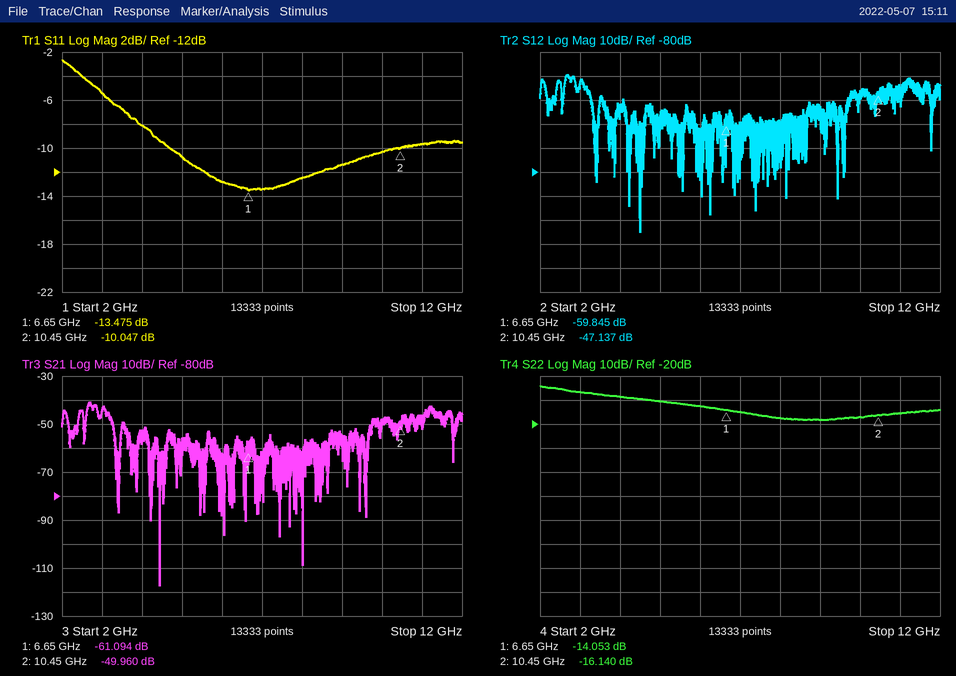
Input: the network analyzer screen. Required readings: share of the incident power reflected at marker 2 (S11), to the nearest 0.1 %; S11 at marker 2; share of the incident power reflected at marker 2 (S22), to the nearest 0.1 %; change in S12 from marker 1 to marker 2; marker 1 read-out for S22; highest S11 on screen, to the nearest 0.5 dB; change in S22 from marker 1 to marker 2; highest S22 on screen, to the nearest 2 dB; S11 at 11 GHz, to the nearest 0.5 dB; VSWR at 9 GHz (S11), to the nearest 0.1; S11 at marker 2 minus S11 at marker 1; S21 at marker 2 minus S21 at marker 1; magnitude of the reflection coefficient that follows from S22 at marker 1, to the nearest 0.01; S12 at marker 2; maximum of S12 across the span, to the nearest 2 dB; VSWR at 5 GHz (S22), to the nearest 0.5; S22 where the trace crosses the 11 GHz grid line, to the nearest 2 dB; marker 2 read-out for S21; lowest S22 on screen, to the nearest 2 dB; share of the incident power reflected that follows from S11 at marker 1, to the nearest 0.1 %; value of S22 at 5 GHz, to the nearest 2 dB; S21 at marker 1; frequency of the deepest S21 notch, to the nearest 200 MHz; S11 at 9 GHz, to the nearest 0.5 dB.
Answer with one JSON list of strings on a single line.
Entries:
["9.9 %", "-10.047 dB", "2.4 %", "12.708 dB", "-14.053 dB", "-2.5 dB", "-2.087 dB", "-4 dB", "-9.5 dB", "1.7", "3.428 dB", "11.134 dB", "0.20", "-47.137 dB", "-40 dB", "2.0", "-16 dB", "-49.960 dB", "-18 dB", "4.5 %", "-10 dB", "-61.094 dB", "4.4 GHz", "-11.5 dB"]
